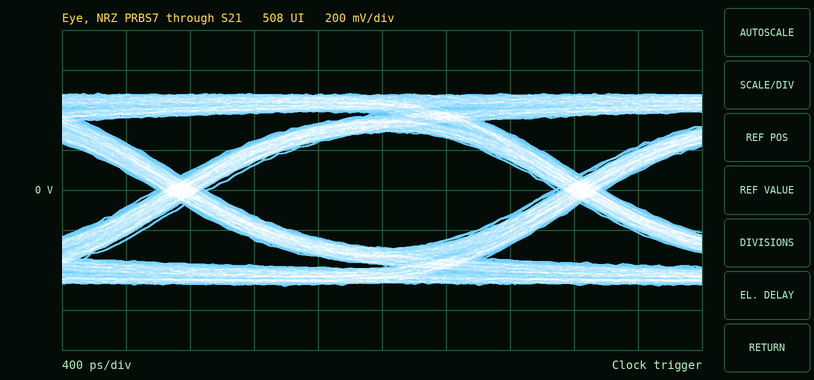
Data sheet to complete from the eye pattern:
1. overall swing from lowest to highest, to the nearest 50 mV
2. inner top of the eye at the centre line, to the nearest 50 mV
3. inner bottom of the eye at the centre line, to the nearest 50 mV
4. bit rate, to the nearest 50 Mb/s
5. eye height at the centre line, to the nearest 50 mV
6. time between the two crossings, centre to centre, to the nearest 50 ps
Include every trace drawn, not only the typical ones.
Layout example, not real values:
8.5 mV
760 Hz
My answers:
950 mV
300 mV
-300 mV
400 Mb/s
600 mV
2.50 ns
